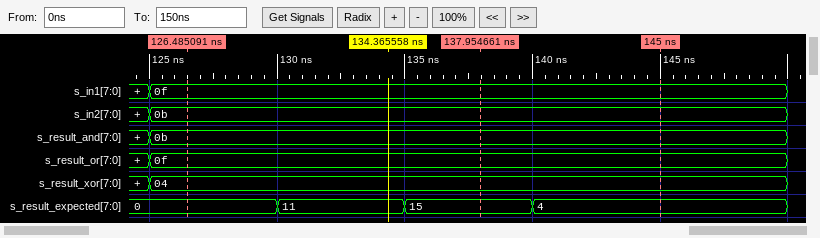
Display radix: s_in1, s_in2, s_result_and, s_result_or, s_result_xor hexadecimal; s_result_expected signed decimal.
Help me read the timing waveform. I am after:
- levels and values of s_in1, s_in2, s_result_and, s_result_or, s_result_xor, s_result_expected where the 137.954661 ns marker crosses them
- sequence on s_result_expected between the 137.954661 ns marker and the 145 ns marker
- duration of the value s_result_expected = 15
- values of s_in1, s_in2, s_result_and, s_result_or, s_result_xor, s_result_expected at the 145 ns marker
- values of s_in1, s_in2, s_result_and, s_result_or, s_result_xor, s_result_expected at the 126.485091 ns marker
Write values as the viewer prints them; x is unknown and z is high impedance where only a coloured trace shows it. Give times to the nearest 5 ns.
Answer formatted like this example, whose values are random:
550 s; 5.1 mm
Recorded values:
s_in1=0f, s_in2=0b, s_result_and=0b, s_result_or=0f, s_result_xor=04, s_result_expected=15; 15, 4; 5 ns; s_in1=0f, s_in2=0b, s_result_and=0b, s_result_or=0f, s_result_xor=04, s_result_expected=4; s_in1=0f, s_in2=0b, s_result_and=0b, s_result_or=0f, s_result_xor=04, s_result_expected=0
